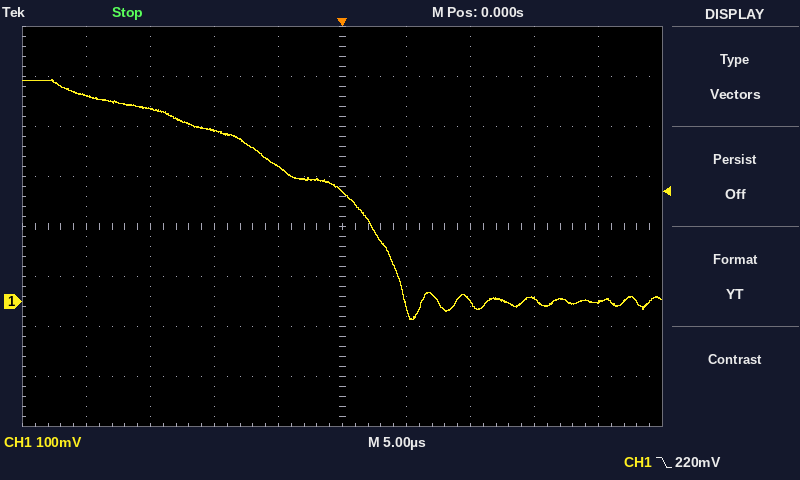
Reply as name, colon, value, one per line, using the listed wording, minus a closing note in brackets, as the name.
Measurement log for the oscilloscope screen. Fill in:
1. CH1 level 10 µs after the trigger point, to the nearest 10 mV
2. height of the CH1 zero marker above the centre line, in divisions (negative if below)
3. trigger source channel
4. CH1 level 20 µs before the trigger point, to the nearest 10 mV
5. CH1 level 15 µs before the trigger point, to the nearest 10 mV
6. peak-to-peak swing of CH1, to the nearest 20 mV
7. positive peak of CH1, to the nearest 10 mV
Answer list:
CH1 level 10 µs after the trigger point, to the nearest 10 mV: 0 mV
height of the CH1 zero marker above the centre line, in divisions: -1.5 div
trigger source channel: CH1
CH1 level 20 µs before the trigger point, to the nearest 10 mV: 410 mV
CH1 level 15 µs before the trigger point, to the nearest 10 mV: 390 mV
peak-to-peak swing of CH1, to the nearest 20 mV: 480 mV
positive peak of CH1, to the nearest 10 mV: 440 mV
